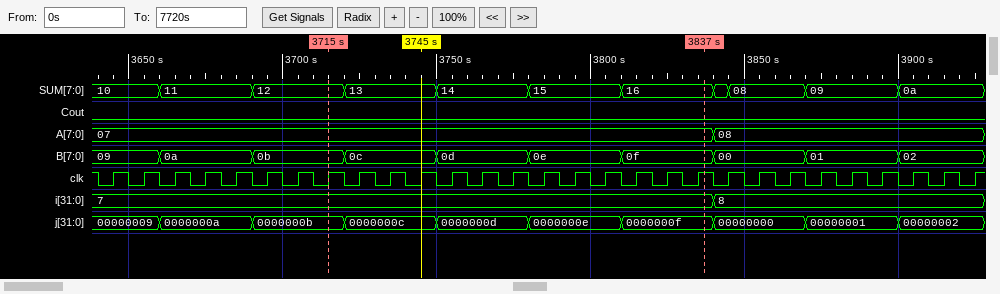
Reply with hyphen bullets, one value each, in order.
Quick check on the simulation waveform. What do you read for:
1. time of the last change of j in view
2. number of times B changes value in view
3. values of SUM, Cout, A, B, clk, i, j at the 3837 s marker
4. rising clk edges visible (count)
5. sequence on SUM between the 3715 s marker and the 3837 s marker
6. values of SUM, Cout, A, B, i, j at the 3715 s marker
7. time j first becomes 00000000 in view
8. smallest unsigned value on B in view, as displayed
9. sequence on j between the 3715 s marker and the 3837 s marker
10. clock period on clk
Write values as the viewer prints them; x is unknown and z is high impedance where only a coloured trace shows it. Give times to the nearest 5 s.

- 3900 s
- 9
- SUM=16, Cout=0, A=07, B=0f, clk=1, i=7, j=0000000f
- 29
- 12, 13, 14, 15, 16
- SUM=12, Cout=0, A=07, B=0b, i=7, j=0000000b
- 3840 s
- 00
- 0000000b, 0000000c, 0000000d, 0000000e, 0000000f
- 10 s
